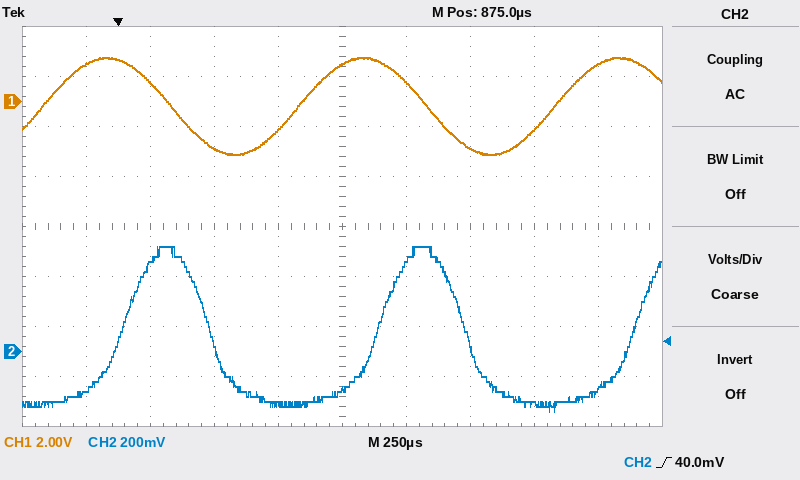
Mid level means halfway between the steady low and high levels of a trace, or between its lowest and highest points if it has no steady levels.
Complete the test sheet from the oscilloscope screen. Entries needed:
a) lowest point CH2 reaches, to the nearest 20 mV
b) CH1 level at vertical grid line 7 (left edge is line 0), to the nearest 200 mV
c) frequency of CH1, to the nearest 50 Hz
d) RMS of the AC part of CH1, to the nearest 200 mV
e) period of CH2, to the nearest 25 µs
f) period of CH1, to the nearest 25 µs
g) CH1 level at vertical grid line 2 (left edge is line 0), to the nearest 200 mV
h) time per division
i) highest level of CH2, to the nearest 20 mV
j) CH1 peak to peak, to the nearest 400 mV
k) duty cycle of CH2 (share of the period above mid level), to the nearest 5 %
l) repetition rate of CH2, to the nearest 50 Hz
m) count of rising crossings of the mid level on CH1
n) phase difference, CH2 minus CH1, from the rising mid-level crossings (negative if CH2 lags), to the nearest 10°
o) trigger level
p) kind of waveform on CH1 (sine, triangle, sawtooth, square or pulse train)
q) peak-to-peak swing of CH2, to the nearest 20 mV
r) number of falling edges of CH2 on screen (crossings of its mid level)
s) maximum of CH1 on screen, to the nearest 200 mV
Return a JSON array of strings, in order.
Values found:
["-240 mV", "-1.8 V", "1.00 kHz", "1.4 V", "1.000 ms", "1.000 ms", "800 mV", "250 µs", "420 mV", "4.0 V", "35 %", "1.00 kHz", "3", "-110°", "40.0 mV", "sine", "660 mV", "2", "1.8 V"]
